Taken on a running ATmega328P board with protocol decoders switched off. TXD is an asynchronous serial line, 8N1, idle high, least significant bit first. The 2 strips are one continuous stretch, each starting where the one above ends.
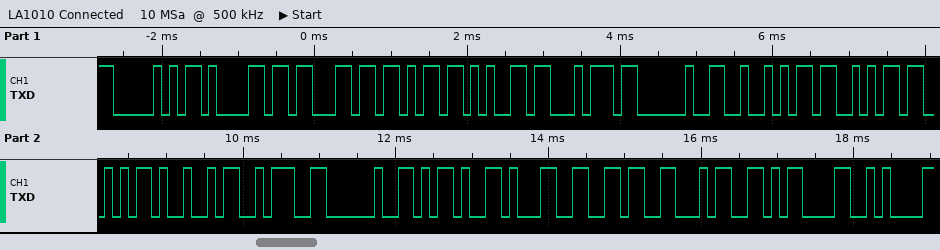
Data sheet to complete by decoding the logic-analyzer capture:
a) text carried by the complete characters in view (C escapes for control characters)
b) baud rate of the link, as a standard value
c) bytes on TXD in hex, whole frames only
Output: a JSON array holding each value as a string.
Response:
["\"Packet RSSI: -164\\r\\n\"", "9600 baud", "50 61 63 6B 65 74 20 52 53 53 49 3A 20 2D 31 36 34 0D 0A"]
